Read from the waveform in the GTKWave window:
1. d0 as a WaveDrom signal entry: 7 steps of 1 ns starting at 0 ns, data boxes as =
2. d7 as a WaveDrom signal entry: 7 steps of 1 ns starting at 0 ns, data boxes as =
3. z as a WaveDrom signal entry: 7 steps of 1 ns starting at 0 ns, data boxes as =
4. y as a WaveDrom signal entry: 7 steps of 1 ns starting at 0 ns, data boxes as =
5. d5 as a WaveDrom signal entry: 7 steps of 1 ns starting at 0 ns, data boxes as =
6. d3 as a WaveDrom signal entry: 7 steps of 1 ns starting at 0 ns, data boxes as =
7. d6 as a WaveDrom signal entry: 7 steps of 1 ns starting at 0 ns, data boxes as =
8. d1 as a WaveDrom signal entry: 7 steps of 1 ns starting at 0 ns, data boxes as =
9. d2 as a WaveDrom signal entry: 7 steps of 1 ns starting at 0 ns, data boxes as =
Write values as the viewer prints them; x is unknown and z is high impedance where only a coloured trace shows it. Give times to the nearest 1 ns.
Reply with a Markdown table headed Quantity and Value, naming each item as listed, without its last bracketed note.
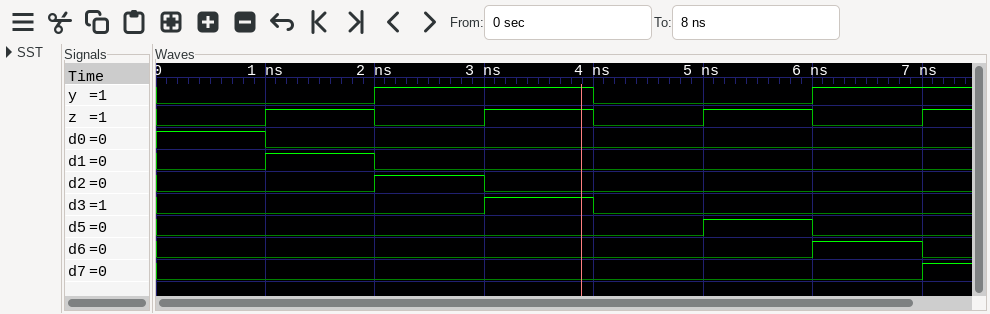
| Quantity | Value |
|---|---|
| d0 as a WaveDrom signal entry: 7 steps of 1 ns starting at 0 ns, data boxes as = | {name: 'd0', wave: '10.....'} |
| d7 as a WaveDrom signal entry: 7 steps of 1 ns starting at 0 ns, data boxes as = | {name: 'd7', wave: '0......'} |
| z as a WaveDrom signal entry: 7 steps of 1 ns starting at 0 ns, data boxes as = | {name: 'z', wave: '0101010'} |
| y as a WaveDrom signal entry: 7 steps of 1 ns starting at 0 ns, data boxes as = | {name: 'y', wave: '0.1.0.1'} |
| d5 as a WaveDrom signal entry: 7 steps of 1 ns starting at 0 ns, data boxes as = | {name: 'd5', wave: '0....10'} |
| d3 as a WaveDrom signal entry: 7 steps of 1 ns starting at 0 ns, data boxes as = | {name: 'd3', wave: '0..10..'} |
| d6 as a WaveDrom signal entry: 7 steps of 1 ns starting at 0 ns, data boxes as = | {name: 'd6', wave: '0.....1'} |
| d1 as a WaveDrom signal entry: 7 steps of 1 ns starting at 0 ns, data boxes as = | {name: 'd1', wave: '010....'} |
| d2 as a WaveDrom signal entry: 7 steps of 1 ns starting at 0 ns, data boxes as = | {name: 'd2', wave: '0.10...'} |
